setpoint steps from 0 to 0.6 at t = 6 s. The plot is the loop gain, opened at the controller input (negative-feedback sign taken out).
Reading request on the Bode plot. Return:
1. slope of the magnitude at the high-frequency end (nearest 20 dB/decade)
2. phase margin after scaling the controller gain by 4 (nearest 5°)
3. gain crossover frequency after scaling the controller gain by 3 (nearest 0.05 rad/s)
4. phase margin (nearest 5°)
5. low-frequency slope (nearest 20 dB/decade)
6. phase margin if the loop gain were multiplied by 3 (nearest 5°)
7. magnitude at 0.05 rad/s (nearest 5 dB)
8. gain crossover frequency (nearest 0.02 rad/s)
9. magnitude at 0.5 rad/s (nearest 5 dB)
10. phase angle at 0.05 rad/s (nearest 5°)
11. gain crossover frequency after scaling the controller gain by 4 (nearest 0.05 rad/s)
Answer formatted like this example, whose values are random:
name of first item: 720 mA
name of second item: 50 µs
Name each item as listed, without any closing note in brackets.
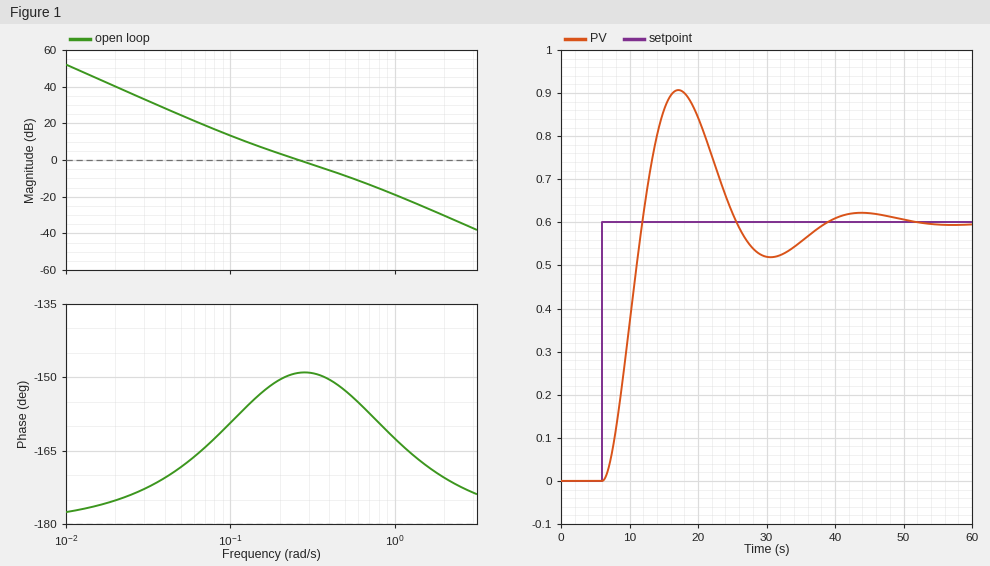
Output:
slope of the magnitude at the high-frequency end: -40 dB/decade
phase margin after scaling the controller gain by 4: 25°
gain crossover frequency after scaling the controller gain by 3: 0.55 rad/s
phase margin: 30°
low-frequency slope: -40 dB/decade
phase margin if the loop gain were multiplied by 3: 25°
magnitude at 0.05 rad/s: 25 dB
gain crossover frequency: 0.26 rad/s
magnitude at 0.5 rad/s: -10 dB
phase angle at 0.05 rad/s: -170°
gain crossover frequency after scaling the controller gain by 4: 0.65 rad/s
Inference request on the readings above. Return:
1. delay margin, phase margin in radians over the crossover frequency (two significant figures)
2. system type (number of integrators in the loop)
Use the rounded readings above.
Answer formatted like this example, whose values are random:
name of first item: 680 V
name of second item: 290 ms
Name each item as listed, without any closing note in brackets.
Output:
delay margin, phase margin in radians over the crossover frequency: 2.0 s
system type: 2
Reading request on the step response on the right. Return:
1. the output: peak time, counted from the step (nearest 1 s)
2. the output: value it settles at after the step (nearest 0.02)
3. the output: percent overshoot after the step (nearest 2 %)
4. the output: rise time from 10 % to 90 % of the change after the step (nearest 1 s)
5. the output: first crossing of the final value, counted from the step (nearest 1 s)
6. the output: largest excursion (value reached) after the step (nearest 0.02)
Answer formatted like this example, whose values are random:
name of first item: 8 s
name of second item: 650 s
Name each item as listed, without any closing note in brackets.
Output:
the output: peak time, counted from the step: 11 s
the output: value it settles at after the step: 0.60
the output: percent overshoot after the step: 52 %
the output: rise time from 10 % to 90 % of the change after the step: 4 s
the output: first crossing of the final value, counted from the step: 6 s
the output: largest excursion (value reached) after the step: 0.90
